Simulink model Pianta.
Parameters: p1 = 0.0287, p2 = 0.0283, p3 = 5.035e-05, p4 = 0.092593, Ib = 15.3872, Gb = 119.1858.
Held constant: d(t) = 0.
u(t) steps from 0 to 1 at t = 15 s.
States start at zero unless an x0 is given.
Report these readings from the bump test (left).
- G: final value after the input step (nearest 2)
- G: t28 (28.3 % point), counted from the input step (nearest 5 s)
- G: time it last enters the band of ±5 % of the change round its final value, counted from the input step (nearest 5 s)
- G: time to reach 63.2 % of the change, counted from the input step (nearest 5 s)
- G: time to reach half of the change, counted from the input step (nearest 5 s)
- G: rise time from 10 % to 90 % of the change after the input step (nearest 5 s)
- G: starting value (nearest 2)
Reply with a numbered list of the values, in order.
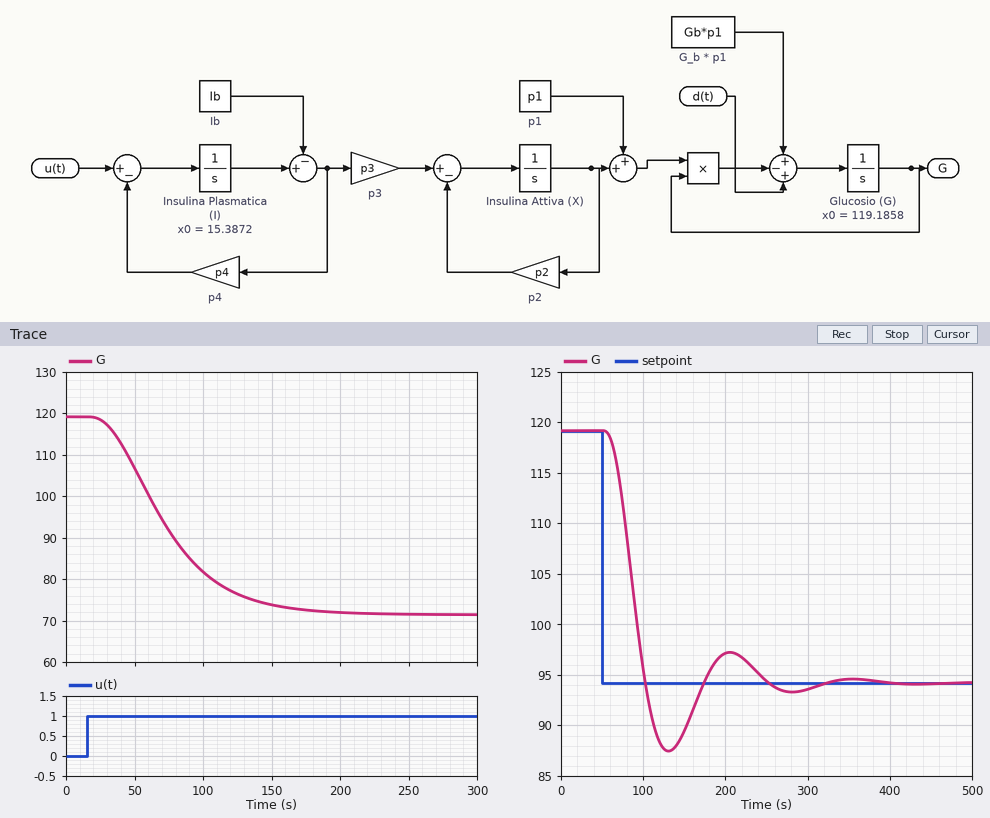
1. 72
2. 35 s
3. 135 s
4. 65 s
5. 55 s
6. 90 s
7. 120
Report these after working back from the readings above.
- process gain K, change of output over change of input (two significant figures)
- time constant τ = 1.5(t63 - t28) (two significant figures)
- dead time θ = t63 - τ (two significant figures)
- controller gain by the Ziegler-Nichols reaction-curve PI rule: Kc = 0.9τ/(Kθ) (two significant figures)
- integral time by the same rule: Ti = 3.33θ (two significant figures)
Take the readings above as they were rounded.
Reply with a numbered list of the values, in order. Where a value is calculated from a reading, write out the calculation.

1. (72 - 120) / 1 = -48
2. 1.5 × (65 - 35) = 45 s
3. 65 - 45 = 20 s
4. 0.9 × 45 / (-48 × 20) = -0.042
5. 3.33 × 20 = 67 s
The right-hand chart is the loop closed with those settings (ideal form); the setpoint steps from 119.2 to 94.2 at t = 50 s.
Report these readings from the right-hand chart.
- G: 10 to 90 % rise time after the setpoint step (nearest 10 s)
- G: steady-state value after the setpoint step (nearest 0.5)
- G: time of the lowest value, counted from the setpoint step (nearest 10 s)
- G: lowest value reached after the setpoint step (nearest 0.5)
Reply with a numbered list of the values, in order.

1. 30 s
2. 94.0
3. 80 s
4. 87.5
